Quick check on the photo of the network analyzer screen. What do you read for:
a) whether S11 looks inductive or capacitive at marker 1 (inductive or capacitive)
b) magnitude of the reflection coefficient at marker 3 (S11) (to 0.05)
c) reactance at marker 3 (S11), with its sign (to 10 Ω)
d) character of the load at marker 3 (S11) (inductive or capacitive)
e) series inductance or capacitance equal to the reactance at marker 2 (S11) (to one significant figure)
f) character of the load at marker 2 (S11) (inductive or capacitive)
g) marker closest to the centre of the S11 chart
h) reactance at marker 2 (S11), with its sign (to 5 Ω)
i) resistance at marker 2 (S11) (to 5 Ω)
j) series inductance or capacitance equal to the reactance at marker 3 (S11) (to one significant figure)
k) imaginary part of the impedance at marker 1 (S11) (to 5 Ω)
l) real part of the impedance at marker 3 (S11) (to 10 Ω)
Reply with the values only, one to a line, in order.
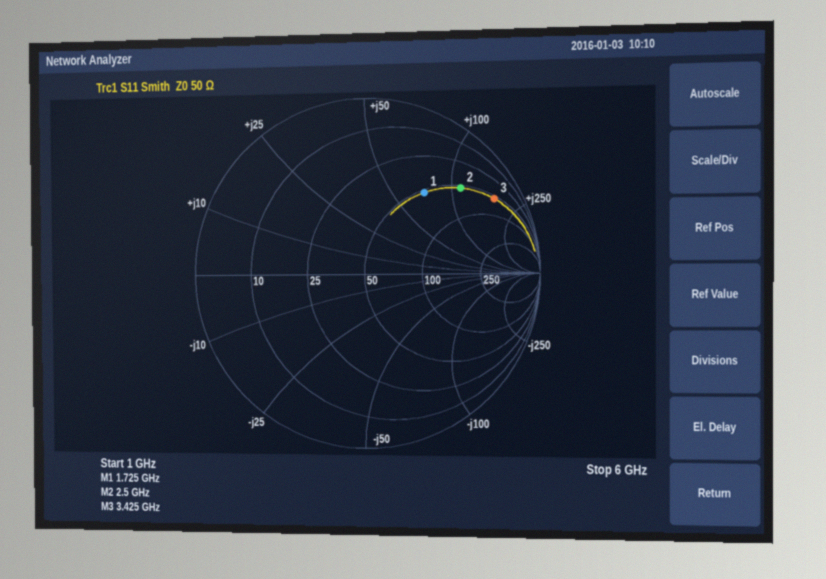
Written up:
inductive
0.85
+170 Ω
inductive
7 nH
inductive
marker 1
+110 Ω
55 Ω
8 nH
+70 Ω
60 Ω
